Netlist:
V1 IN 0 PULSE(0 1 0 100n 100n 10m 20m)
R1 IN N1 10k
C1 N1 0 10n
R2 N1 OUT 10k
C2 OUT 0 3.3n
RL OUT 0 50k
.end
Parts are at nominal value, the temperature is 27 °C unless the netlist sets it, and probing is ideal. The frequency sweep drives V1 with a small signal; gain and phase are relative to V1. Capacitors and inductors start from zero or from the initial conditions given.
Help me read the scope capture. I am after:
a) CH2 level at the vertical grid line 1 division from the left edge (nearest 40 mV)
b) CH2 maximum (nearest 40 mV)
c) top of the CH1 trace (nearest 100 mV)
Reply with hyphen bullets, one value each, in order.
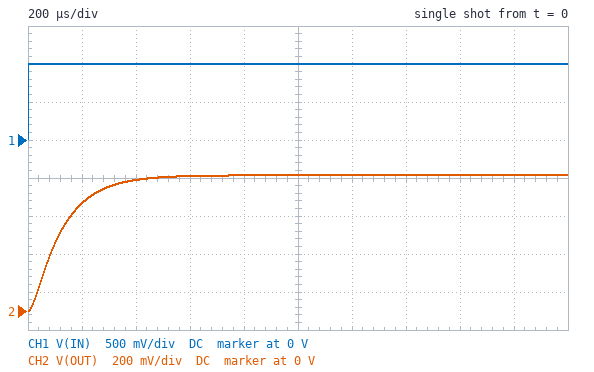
- 560 mV
- 720 mV
- 1.0 V
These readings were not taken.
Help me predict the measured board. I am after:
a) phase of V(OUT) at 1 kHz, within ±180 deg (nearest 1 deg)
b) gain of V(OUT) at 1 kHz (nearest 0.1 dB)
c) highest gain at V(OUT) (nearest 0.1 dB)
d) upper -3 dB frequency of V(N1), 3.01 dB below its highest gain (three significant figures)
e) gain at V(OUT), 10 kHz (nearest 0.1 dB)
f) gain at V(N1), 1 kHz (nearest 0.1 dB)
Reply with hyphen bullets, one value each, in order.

- -43 deg
- -4.7 dB
- -2.9 dB
- 1.46 kHz
- -24.3 dB
- -3.0 dB
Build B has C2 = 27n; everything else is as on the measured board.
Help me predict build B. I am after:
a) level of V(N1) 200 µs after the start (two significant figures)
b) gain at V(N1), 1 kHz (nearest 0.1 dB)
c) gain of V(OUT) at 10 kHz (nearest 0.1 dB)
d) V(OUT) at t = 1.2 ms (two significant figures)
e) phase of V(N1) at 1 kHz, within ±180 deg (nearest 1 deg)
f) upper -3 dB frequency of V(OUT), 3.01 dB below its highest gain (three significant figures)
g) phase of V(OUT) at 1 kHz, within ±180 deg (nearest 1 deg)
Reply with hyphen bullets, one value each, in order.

- 570 mV
- -6.0 dB
- -41.1 dB
- 670 mV
- -31 deg
- 369 Hz
- -85 deg
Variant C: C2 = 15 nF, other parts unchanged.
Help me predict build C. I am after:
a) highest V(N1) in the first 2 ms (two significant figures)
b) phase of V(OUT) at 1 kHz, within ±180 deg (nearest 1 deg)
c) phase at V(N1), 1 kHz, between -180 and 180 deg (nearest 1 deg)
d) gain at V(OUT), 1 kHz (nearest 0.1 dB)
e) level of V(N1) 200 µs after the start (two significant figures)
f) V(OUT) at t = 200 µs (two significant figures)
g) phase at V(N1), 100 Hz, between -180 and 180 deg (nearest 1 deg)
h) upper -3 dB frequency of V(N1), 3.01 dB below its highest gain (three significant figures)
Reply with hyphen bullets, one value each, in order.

- 860 mV
- -73 deg
- -35 deg
- -8.8 dB
- 610 mV
- 320 mV
- -6 deg
- 794 Hz
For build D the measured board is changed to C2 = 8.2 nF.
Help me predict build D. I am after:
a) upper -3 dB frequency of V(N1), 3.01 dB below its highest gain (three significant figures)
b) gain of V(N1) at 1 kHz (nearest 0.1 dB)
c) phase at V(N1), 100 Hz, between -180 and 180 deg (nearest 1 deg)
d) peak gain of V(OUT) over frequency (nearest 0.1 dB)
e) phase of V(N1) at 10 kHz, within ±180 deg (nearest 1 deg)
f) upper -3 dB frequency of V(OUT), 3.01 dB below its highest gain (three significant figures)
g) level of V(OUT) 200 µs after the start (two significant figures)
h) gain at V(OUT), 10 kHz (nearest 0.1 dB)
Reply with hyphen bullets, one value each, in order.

- 1.08 kHz
- -4.1 dB
- -5 deg
- -2.9 dB
- -73 deg
- 910 Hz
- 440 mV
- -31.1 dB
